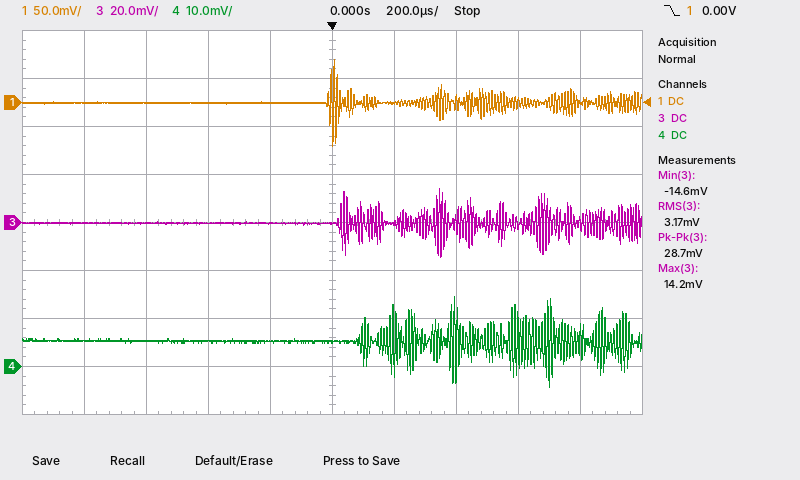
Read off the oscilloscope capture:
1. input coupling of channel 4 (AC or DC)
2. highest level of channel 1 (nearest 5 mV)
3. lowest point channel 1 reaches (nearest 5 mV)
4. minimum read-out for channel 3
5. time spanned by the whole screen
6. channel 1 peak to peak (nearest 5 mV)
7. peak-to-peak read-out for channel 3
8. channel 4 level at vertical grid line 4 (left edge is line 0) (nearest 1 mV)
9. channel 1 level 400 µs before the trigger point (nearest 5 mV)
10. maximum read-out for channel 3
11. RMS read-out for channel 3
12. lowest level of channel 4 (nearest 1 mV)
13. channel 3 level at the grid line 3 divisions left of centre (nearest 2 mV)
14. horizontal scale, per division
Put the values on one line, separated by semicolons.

DC; 45 mV; -45 mV; -14.6 mV; 2 ms; 90 mV; 28.7 mV; 5 mV; 0 mV; 14.2 mV; 3.17 mV; -4 mV; 0 mV; 200 µs
